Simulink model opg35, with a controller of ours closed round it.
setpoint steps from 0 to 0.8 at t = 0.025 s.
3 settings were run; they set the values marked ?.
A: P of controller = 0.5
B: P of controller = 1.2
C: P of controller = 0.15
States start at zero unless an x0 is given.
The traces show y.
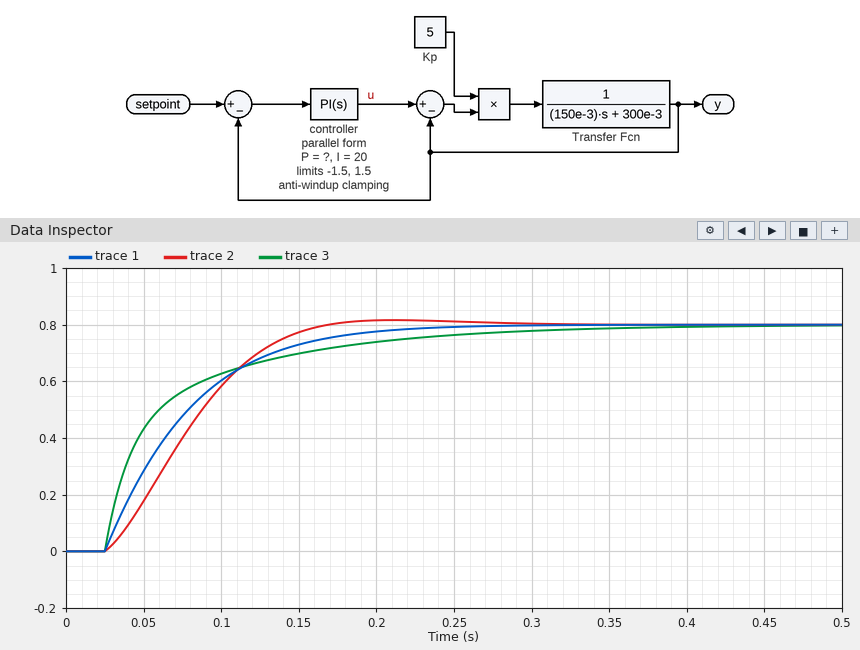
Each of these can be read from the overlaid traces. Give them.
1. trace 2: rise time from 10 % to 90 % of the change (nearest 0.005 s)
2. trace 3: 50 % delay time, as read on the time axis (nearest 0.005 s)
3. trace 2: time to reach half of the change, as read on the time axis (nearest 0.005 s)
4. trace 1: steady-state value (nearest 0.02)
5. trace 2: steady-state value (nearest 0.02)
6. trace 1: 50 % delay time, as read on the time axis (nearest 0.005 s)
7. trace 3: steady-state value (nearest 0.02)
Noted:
0.090 s
0.045 s
0.075 s
0.80
0.80
0.065 s
0.80
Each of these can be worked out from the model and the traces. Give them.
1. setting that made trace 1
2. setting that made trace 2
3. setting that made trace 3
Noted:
A
C
B
